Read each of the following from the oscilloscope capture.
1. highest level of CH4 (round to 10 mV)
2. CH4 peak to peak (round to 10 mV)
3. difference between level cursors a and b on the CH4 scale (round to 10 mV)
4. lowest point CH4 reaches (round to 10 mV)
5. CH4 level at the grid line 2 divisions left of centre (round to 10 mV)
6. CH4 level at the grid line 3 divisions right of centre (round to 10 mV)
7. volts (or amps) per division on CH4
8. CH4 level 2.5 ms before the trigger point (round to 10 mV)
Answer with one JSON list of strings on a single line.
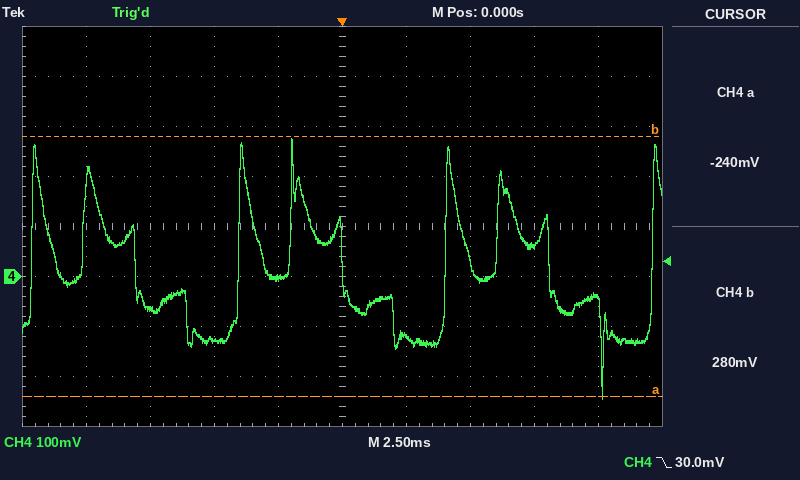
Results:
["280 mV", "520 mV", "520 mV", "-240 mV", "-130 mV", "60 mV", "100 mV", "0 mV"]
